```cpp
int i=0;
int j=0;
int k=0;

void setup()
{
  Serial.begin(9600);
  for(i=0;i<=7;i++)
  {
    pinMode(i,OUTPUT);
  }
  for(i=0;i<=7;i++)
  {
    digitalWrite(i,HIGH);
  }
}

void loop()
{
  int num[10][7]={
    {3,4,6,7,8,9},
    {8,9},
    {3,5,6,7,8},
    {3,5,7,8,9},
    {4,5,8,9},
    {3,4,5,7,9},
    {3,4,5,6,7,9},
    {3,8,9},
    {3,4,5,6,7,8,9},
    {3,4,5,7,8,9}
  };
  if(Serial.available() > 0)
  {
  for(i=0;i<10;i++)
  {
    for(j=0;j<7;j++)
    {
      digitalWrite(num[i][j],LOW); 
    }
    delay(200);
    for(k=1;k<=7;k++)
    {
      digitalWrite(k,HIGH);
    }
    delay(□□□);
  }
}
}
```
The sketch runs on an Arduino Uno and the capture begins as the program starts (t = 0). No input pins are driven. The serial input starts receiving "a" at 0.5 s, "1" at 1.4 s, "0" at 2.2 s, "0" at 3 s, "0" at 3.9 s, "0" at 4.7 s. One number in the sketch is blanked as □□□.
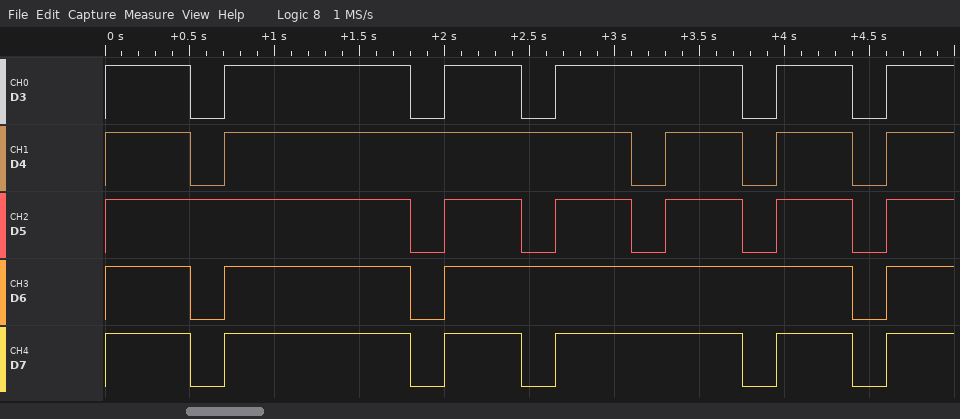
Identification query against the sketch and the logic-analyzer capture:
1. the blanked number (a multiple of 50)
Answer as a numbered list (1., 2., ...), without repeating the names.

1. 450
